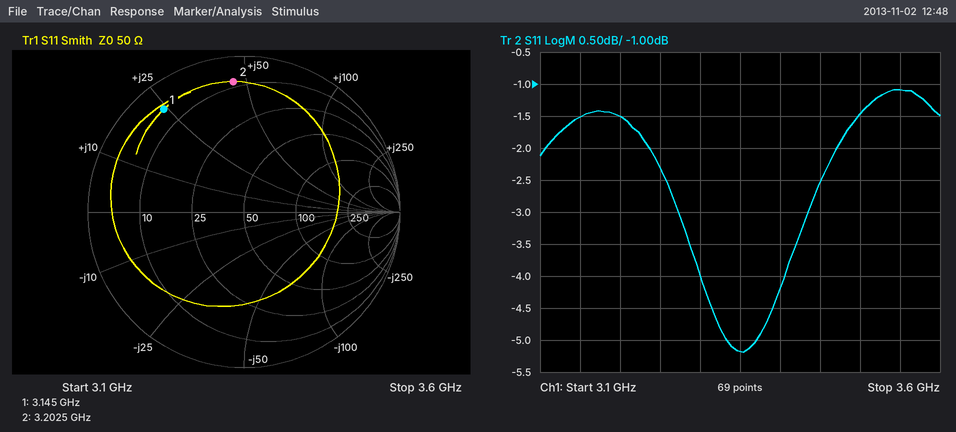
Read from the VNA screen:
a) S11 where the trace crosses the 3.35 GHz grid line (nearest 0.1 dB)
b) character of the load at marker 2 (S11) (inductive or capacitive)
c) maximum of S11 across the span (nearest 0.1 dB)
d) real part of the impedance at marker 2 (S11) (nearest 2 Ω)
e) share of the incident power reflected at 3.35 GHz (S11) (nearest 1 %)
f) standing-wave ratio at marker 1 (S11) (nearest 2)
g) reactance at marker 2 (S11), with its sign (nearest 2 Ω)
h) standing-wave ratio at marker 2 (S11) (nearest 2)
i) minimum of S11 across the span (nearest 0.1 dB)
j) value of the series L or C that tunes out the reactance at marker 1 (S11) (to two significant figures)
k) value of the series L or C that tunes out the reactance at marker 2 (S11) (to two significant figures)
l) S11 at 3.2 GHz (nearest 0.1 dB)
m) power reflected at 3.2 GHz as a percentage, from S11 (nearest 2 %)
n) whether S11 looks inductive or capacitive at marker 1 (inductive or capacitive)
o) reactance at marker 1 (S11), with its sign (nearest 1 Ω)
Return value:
-5.2 dB
inductive
-1.1 dB
8 Ω
30 %
12
+46 Ω
12
-5.2 dB
2.1 pF
1.1 pF
-1.5 dB
70 %
inductive
+24 Ω
